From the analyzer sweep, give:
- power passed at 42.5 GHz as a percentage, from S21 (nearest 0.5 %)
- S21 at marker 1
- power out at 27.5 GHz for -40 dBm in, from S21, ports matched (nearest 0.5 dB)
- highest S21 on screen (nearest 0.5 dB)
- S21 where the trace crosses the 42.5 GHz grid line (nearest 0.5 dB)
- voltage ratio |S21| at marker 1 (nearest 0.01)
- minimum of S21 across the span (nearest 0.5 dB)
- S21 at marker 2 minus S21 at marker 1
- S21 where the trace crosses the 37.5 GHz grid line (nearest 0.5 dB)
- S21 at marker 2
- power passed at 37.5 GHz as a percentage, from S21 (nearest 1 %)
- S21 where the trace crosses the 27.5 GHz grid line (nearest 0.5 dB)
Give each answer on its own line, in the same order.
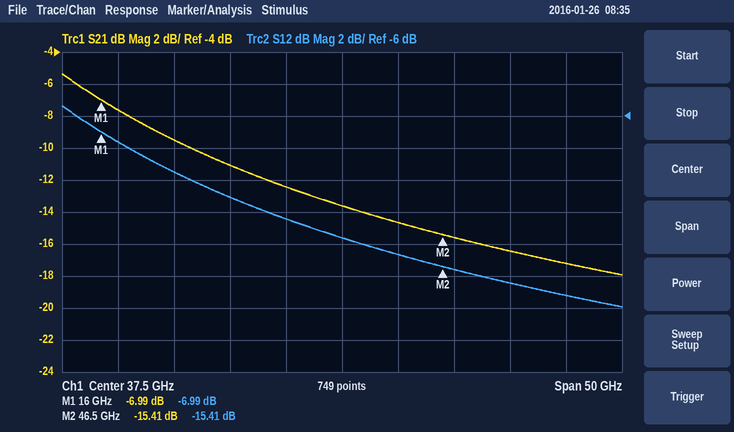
3.5 %
-6.99 dB
-51.0 dBm
-5.5 dB
-14.5 dB
0.45
-18.0 dB
-8.42 dB
-13.5 dB
-15.41 dB
4 %
-11.0 dB
